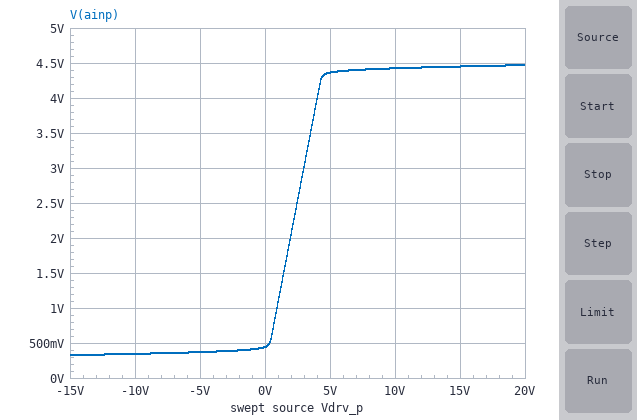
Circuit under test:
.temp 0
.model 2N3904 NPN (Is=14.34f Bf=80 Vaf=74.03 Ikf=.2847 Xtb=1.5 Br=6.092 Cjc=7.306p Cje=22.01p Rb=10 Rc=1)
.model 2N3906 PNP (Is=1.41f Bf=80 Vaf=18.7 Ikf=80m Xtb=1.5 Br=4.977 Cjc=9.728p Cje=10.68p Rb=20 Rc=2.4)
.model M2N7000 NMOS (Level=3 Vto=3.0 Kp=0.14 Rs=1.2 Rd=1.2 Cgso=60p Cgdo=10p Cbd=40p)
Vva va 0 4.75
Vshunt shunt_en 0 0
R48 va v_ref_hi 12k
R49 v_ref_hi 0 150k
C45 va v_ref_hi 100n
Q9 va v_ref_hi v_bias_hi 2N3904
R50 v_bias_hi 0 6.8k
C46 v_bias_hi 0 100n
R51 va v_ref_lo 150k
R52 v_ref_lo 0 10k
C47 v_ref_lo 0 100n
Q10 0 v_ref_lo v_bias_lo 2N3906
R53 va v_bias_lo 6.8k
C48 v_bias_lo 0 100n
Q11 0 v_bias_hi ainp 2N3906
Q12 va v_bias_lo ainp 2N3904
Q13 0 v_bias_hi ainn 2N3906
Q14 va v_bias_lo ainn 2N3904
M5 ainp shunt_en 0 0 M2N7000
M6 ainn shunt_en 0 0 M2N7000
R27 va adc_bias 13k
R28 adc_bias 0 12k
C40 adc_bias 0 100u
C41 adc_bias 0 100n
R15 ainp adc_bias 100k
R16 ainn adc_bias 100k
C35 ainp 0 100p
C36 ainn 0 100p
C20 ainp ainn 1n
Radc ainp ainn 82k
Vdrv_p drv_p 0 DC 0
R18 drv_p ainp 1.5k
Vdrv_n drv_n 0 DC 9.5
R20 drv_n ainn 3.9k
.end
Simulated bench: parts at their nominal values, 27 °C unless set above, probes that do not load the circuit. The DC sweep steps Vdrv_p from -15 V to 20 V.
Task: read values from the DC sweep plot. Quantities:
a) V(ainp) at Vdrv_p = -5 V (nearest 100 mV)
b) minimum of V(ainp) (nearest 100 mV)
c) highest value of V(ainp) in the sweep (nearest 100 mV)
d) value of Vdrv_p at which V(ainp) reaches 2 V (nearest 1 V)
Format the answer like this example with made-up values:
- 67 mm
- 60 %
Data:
- 400 mV
- 300 mV
- 4.5 V
- 2 V
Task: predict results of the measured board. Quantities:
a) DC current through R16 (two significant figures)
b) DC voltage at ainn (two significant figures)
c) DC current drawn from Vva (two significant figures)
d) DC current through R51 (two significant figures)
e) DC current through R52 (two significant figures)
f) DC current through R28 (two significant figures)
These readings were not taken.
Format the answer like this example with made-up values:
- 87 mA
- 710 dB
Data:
- 21 µA
- 4.4 V
- 1.5 mA
- 29 µA
- 37 µA
- 190 µA
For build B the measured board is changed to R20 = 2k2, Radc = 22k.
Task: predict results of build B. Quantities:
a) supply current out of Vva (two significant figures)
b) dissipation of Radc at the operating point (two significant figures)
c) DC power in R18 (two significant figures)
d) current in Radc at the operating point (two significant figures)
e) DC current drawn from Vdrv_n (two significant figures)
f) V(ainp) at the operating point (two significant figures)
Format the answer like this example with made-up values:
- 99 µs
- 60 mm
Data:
- 1.4 mA
- 710 µW
- 140 µW
- 180 µA
- 2.3 mA
- 460 mV
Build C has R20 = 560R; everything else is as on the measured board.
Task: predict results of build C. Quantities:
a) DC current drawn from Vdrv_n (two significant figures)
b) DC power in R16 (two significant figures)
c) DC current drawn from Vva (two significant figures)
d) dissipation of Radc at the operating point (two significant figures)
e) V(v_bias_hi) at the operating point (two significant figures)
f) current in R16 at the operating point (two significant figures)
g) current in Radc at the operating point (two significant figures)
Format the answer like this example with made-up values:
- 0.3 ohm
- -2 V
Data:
- 9.0 mA
- 47 µW
- 1.4 mA
- 200 µW
- 3.7 V
- 22 µA
- 49 µA
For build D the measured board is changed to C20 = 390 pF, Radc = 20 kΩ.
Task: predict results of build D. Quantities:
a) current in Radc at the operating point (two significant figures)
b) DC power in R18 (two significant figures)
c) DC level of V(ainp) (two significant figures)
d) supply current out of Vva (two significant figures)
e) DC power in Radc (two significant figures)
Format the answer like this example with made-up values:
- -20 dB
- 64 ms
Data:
- 200 µA
- 140 µW
- 460 mV
- 1.4 mA
- 770 µW
